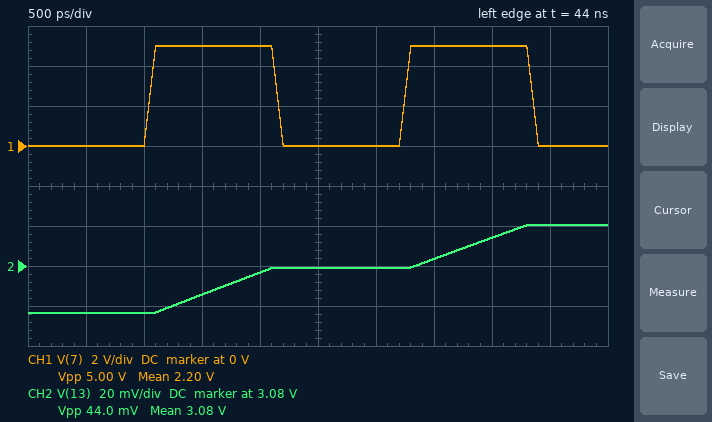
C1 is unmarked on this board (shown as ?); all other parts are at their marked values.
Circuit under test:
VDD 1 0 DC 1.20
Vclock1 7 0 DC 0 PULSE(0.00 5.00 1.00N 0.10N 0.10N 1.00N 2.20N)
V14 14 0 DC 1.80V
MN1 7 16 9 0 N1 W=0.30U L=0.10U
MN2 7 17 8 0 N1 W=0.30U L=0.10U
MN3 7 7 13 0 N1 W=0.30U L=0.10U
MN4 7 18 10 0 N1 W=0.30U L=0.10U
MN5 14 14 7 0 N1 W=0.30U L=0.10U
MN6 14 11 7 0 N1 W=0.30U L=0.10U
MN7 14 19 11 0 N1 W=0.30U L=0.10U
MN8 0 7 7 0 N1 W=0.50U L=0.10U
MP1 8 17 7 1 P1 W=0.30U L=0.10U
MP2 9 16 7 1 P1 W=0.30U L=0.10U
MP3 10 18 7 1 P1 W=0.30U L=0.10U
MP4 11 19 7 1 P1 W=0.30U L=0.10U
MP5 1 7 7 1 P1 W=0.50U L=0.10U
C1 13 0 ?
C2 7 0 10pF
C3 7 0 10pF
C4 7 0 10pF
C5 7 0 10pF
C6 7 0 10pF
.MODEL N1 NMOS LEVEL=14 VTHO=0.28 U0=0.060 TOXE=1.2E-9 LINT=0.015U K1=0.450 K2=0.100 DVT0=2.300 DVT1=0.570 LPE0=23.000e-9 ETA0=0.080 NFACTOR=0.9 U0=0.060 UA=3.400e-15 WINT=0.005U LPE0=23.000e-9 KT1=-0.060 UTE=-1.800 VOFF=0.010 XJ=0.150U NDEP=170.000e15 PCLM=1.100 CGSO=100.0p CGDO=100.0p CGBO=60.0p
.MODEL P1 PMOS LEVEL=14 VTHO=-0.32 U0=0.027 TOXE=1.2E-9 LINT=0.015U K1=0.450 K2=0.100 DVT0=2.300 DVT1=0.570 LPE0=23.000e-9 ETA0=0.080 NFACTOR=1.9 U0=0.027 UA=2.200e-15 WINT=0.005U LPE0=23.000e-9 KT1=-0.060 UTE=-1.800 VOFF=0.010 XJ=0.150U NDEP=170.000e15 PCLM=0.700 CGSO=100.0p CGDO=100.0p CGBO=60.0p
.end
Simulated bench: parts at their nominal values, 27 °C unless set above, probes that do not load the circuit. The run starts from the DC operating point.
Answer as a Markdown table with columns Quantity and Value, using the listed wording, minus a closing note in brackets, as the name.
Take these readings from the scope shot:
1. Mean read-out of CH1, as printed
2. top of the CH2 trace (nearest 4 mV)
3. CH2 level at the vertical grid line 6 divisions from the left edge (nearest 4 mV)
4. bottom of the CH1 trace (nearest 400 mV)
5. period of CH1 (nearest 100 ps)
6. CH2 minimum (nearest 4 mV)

| Quantity | Value |
|---|---|
| Mean read-out of CH1, as printed | 2.20 V |
| top of the CH2 trace | 3.100 V |
| CH2 level at the vertical grid line 6 divisions from the left edge | 3.080 V |
| bottom of the CH1 trace | 0 V |
| period of CH1 | 2.2 ns |
| CH2 minimum | 3.056 V |
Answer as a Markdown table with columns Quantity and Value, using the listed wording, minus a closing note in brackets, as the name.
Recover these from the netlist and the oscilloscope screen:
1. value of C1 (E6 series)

| Quantity | Value |
|---|---|
| value of C1 | 33 pF |
